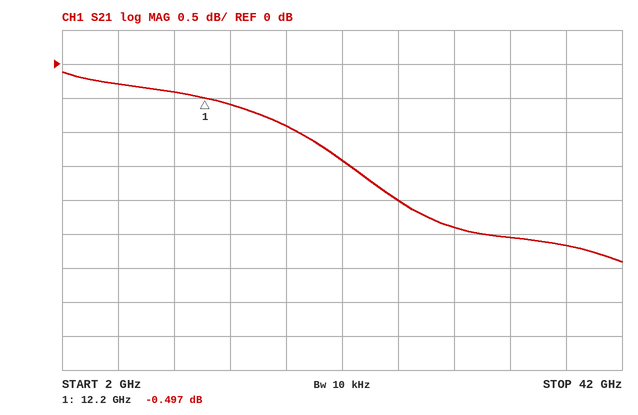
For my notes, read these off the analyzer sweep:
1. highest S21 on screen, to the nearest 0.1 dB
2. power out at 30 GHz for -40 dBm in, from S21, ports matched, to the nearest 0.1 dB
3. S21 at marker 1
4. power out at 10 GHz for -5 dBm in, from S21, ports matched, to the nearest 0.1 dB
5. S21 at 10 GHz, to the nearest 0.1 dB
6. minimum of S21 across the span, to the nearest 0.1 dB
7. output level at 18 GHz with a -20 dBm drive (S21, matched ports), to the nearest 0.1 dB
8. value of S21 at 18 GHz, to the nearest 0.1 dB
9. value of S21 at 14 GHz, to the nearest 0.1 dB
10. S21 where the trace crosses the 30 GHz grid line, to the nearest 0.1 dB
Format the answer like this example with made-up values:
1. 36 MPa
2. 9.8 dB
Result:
1. -0.1 dB
2. -42.4 dBm
3. -0.497 dB
4. -5.4 dBm
5. -0.4 dB
6. -2.9 dB
7. -20.9 dBm
8. -0.9 dB
9. -0.6 dB
10. -2.4 dB
